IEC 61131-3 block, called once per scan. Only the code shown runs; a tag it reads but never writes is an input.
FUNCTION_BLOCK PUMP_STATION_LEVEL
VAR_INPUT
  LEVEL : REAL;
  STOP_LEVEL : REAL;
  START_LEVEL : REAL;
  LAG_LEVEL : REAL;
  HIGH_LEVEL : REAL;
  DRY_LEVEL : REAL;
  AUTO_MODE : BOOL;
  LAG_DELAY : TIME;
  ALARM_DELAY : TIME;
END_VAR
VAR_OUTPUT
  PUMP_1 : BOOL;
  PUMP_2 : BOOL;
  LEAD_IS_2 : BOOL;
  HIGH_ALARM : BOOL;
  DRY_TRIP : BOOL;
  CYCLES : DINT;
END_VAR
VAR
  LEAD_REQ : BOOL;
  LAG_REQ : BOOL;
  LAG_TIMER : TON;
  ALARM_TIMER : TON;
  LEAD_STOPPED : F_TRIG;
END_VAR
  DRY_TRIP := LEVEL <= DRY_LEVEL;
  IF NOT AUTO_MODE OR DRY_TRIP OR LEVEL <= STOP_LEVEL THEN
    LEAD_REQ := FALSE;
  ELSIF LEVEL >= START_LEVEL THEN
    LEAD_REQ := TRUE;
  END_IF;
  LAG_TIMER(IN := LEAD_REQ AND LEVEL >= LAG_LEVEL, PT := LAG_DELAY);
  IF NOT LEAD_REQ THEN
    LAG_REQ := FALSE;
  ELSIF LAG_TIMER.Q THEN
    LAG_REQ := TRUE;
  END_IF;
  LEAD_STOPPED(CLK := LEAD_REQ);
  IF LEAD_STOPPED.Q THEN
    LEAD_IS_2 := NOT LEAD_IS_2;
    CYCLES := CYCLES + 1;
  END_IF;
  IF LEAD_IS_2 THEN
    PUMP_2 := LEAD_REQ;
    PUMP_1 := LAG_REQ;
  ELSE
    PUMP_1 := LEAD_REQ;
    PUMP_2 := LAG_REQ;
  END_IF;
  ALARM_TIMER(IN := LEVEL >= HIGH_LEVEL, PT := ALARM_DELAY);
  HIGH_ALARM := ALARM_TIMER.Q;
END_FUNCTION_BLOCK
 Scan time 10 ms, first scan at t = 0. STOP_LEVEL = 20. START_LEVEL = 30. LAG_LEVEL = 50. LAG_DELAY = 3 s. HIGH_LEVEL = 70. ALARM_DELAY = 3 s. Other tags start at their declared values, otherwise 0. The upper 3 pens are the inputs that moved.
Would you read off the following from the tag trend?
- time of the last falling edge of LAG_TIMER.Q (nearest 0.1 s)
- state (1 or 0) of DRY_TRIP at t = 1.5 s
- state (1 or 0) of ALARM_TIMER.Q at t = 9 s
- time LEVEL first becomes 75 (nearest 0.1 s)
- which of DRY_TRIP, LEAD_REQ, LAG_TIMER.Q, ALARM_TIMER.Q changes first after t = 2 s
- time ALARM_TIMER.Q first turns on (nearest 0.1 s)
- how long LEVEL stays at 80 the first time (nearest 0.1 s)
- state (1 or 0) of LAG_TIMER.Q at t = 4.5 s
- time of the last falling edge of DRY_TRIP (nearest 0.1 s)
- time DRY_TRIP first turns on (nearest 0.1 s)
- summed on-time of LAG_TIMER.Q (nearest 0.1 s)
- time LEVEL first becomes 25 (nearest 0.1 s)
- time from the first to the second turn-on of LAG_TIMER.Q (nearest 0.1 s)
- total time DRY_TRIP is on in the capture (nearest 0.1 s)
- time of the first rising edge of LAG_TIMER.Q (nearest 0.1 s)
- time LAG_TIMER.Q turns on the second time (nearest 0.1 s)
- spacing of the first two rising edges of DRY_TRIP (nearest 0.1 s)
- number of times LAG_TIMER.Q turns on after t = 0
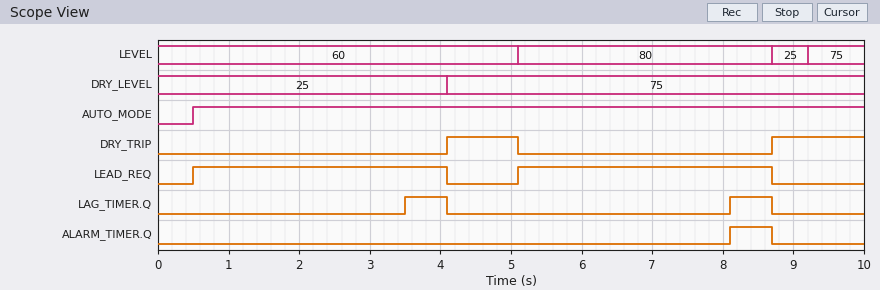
8.7 s
0
0
9.2 s
LAG_TIMER.Q
8.1 s
3.6 s
0
5.1 s
4.1 s
1.2 s
8.7 s
4.6 s
2.3 s
3.5 s
8.1 s
4.6 s
2
